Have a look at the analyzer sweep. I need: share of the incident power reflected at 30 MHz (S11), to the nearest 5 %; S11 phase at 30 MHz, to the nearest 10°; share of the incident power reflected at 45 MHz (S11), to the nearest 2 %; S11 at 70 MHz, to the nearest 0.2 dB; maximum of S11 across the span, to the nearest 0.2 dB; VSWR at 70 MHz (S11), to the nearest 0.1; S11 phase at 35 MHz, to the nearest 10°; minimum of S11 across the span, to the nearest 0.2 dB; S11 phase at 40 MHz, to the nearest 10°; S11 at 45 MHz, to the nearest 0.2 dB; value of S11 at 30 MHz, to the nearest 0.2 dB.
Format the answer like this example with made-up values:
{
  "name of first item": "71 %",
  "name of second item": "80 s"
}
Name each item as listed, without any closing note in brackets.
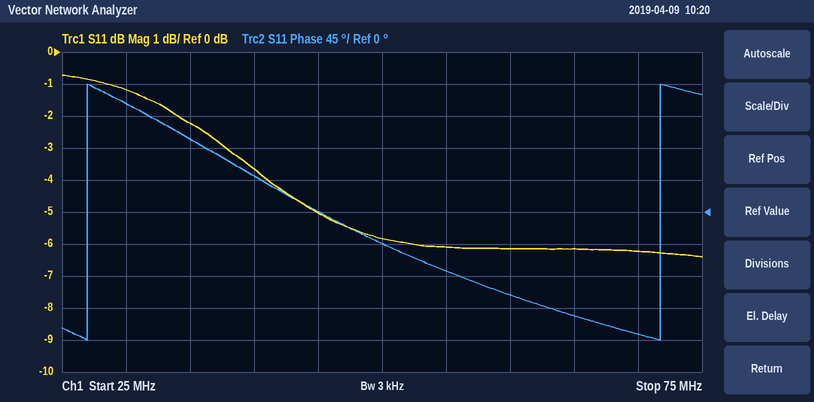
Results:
{
  "share of the incident power reflected at 30 MHz (S11), to the nearest 5 %": "75 %",
  "S11 phase at 30 MHz, to the nearest 10°": "150°",
  "share of the incident power reflected at 45 MHz (S11), to the nearest 2 %": "32 %",
  "S11 at 70 MHz, to the nearest 0.2 dB": "-6.2 dB",
  "maximum of S11 across the span, to the nearest 0.2 dB": "-0.8 dB",
  "VSWR at 70 MHz (S11), to the nearest 0.1": "2.9",
  "S11 phase at 35 MHz, to the nearest 10°": "100°",
  "minimum of S11 across the span, to the nearest 0.2 dB": "-6.4 dB",
  "S11 phase at 40 MHz, to the nearest 10°": "50°",
  "S11 at 45 MHz, to the nearest 0.2 dB": "-5.0 dB",
  "value of S11 at 30 MHz, to the nearest 0.2 dB": "-1.2 dB"
}
